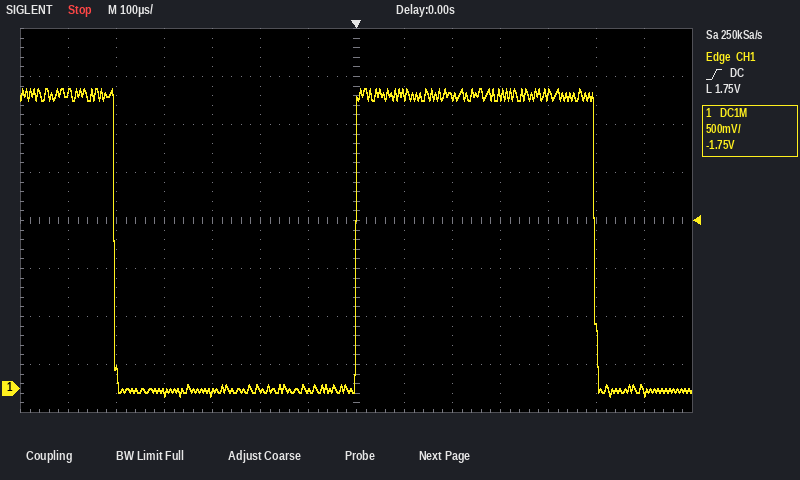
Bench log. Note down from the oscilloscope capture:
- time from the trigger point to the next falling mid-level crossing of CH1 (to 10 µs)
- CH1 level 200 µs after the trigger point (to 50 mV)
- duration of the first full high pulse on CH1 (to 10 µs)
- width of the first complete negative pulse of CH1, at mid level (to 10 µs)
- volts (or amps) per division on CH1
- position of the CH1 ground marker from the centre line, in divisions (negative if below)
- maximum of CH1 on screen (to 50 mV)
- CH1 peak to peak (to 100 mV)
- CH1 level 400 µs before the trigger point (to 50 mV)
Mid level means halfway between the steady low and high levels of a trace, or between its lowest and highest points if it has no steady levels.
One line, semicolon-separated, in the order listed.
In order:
500 µs; 3.05 V; 500 µs; 500 µs; 500 mV; -3.5 div; 3.10 V; 3.20 V; -50 mV
